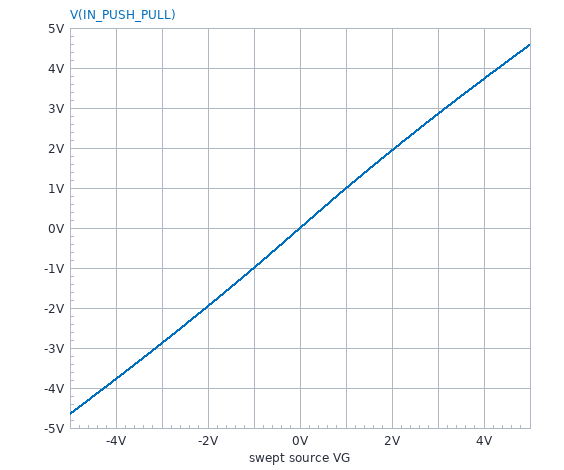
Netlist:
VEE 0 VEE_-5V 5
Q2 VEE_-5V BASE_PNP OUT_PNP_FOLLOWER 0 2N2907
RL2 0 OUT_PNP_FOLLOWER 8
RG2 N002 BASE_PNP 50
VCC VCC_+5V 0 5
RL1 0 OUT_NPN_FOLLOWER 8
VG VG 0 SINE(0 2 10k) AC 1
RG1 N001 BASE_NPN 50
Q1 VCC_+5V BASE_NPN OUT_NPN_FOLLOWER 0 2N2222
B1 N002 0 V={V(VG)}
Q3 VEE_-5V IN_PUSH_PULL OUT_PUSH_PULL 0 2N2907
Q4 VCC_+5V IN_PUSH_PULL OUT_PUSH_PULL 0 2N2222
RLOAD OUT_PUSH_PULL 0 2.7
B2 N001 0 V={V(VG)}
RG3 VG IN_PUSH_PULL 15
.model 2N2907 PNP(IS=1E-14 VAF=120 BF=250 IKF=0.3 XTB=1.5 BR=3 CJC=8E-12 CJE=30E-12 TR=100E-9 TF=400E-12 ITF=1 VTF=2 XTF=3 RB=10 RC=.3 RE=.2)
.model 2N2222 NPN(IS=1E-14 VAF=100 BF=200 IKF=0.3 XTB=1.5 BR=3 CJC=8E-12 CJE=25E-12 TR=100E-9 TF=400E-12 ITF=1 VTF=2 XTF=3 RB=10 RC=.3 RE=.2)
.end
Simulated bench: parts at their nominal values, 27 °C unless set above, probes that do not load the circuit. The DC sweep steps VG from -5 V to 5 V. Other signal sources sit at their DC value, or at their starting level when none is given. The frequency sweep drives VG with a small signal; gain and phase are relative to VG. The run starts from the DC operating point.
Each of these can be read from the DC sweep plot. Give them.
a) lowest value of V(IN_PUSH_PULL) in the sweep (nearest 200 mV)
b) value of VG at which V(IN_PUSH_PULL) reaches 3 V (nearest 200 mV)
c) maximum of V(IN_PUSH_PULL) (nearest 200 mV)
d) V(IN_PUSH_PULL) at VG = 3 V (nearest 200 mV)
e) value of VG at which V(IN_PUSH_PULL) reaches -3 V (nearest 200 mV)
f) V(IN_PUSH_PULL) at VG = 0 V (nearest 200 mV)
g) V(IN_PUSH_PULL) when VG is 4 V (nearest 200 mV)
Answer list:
-4.6 V
3.2 V
4.6 V
2.8 V
-3.2 V
0 V
3.8 V
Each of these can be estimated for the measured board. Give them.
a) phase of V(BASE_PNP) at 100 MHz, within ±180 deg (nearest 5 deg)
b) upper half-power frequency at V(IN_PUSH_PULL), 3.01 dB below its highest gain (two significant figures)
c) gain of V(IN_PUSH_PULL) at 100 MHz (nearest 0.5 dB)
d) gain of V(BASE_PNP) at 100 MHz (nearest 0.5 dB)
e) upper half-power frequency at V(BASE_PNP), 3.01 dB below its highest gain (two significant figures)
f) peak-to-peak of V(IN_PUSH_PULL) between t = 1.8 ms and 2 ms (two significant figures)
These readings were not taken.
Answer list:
-35 deg
130 MHz
-2.0 dB
-4.5 dB
75 MHz
3.9 V
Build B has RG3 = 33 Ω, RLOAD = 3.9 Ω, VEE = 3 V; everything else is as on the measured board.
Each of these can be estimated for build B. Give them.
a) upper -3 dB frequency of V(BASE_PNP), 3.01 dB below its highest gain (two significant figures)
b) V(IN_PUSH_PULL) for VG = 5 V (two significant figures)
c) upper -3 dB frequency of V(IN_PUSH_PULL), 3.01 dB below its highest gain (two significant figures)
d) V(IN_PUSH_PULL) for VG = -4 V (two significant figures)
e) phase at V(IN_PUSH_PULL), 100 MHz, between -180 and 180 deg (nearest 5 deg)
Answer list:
74 MHz
4.5 V
63 MHz
-3.6 V
-40 deg
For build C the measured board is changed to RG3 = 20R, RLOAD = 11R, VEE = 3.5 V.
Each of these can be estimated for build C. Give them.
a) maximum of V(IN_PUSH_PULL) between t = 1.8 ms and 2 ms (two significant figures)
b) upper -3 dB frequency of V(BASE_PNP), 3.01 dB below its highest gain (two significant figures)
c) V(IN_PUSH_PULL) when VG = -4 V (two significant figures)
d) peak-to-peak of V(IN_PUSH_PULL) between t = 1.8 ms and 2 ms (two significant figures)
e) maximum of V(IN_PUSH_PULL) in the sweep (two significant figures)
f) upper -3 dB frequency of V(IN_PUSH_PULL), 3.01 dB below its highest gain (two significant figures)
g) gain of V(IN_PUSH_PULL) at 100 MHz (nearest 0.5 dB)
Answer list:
2.0 V
74 MHz
-4.0 V
4.0 V
4.9 V
92 MHz
-3.5 dB
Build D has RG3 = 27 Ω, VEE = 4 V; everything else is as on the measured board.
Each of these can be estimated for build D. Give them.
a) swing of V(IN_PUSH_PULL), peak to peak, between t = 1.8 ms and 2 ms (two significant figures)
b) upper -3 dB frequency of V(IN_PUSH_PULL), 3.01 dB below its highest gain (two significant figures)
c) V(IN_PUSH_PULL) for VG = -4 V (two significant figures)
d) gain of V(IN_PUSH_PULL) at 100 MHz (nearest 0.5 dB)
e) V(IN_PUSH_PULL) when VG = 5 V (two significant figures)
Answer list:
3.8 V
77 MHz
-3.6 V
-4.0 dB
4.3 V
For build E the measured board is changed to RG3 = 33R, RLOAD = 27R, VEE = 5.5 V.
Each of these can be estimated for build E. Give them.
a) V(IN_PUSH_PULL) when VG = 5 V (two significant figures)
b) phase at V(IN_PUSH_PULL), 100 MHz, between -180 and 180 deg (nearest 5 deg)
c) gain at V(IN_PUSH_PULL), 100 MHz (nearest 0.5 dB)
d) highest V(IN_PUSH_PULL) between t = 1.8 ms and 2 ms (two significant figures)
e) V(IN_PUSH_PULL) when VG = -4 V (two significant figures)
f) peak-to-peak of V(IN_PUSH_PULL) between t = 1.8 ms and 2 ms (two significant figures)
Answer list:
5.0 V
-20 deg
-4.5 dB
2.0 V
-4.0 V
4.0 V
